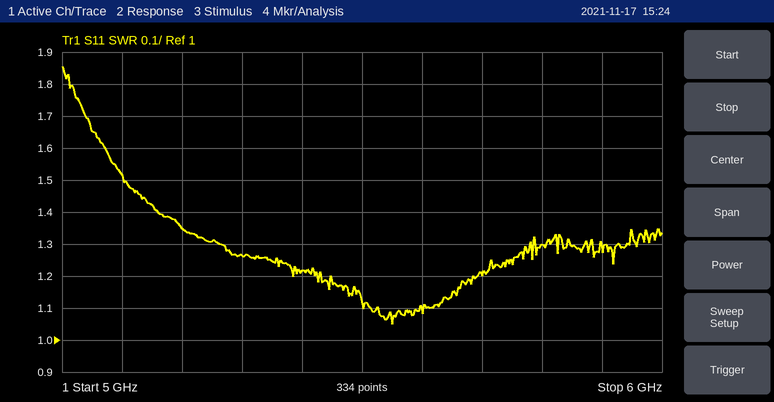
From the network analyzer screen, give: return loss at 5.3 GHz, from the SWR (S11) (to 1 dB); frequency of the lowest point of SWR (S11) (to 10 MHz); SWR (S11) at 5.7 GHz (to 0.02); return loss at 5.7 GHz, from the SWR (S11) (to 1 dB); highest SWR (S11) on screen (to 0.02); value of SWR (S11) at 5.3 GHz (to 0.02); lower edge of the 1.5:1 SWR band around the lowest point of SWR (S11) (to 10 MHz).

19 dB
5.55 GHz
1.20
21 dB
1.86
1.26
5.10 GHz
